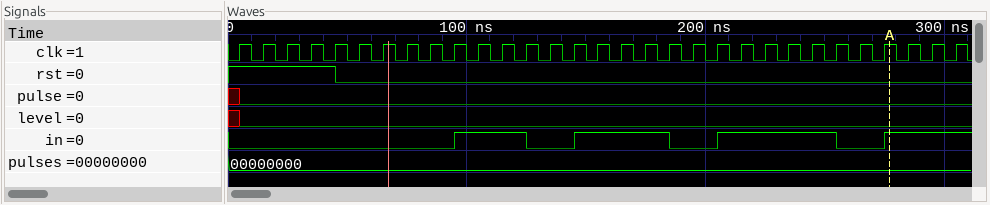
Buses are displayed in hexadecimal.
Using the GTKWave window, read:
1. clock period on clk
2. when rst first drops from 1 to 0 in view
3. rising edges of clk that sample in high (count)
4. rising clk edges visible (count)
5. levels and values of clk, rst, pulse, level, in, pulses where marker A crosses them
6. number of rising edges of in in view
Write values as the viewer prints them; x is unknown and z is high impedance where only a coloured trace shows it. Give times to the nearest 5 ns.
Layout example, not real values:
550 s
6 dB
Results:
10 ns
45 ns
15
31
clk=1, rst=0, pulse=0, level=0, in=1, pulses=00000000
4
